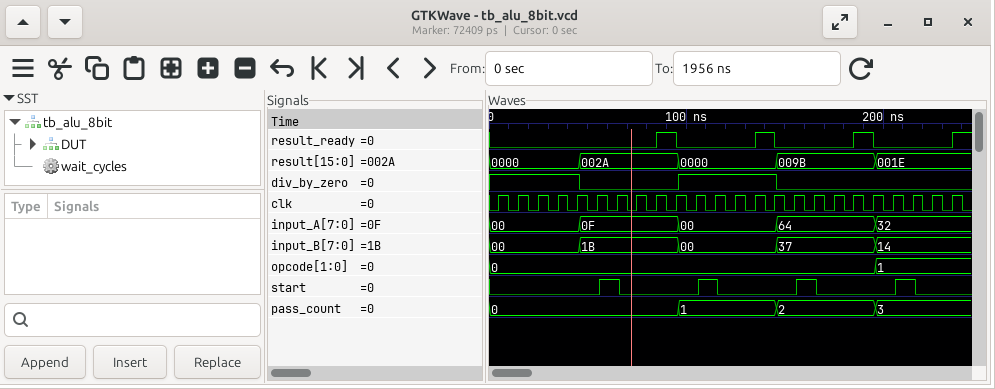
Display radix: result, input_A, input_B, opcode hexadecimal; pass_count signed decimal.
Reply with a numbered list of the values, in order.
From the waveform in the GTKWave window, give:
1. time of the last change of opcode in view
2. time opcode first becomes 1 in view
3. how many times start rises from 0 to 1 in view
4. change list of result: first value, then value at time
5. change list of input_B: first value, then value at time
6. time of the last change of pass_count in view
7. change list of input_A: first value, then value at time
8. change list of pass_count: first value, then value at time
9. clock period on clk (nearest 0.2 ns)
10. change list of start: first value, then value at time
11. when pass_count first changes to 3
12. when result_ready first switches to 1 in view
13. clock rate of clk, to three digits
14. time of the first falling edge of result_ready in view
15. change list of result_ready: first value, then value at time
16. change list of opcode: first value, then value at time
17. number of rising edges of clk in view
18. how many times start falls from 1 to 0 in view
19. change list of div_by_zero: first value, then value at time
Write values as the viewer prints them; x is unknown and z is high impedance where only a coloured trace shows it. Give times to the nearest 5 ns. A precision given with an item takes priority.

1. 195 ns
2. 195 ns
3. 4
4. 0000, 002A at 45 ns, 0000 at 95 ns, 009B at 145 ns, 001E at 195 ns
5. 00, 1B at 45 ns, 00 at 95 ns, 37 at 145 ns, 14 at 195 ns
6. 195 ns
7. 00, 0F at 45 ns, 00 at 95 ns, 64 at 145 ns, 32 at 195 ns
8. 0, 1 at 95 ns, 2 at 145 ns, 3 at 195 ns
9. 10 ns
10. 0, 1 at 55 ns, 0 at 65 ns, 1 at 105 ns, 0 at 115 ns, 1 at 155 ns, 0 at 165 ns, 1 at 205 ns, 0 at 215 ns
11. 195 ns
12. 85 ns
13. 100 MHz
14. 95 ns
15. 0, 1 at 85 ns, 0 at 95 ns, 1 at 135 ns, 0 at 145 ns, 1 at 185 ns, 0 at 195 ns, 1 at 235 ns
16. 0, 1 at 195 ns
17. 24
18. 4
19. 1, 0 at 45 ns, 1 at 95 ns, 0 at 145 ns
